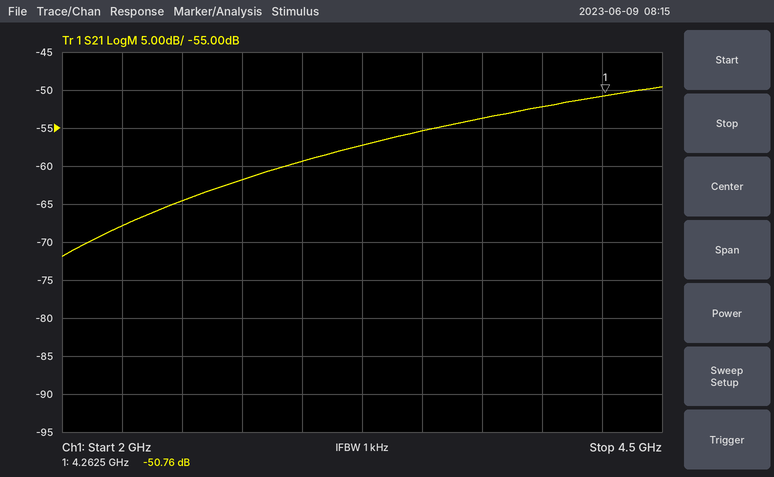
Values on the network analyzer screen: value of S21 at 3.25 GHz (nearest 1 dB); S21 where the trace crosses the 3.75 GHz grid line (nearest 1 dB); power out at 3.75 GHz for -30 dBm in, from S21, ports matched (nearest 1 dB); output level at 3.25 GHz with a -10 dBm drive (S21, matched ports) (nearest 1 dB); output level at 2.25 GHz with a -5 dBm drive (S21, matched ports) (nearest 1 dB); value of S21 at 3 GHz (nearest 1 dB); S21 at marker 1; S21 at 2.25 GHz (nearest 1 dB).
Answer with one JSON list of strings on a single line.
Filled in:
["-57 dB", "-54 dB", "-84 dBm", "-67 dBm", "-73 dBm", "-59 dB", "-50.76 dB", "-68 dB"]
